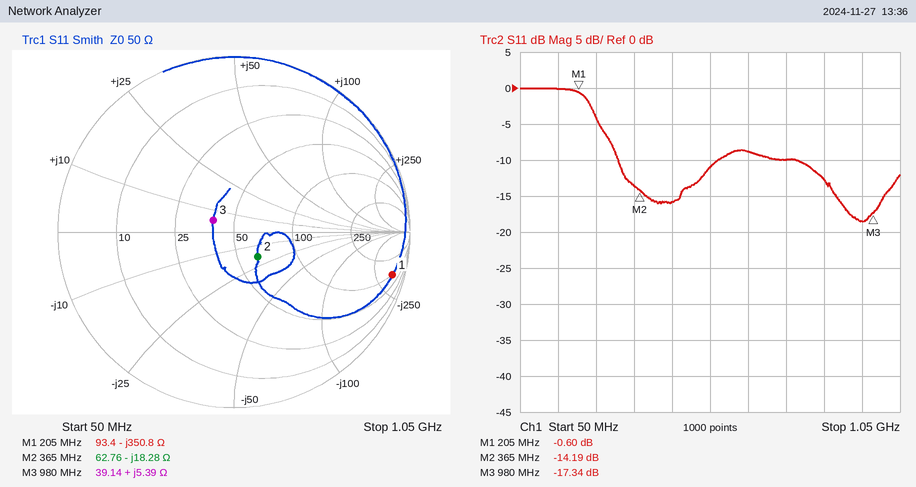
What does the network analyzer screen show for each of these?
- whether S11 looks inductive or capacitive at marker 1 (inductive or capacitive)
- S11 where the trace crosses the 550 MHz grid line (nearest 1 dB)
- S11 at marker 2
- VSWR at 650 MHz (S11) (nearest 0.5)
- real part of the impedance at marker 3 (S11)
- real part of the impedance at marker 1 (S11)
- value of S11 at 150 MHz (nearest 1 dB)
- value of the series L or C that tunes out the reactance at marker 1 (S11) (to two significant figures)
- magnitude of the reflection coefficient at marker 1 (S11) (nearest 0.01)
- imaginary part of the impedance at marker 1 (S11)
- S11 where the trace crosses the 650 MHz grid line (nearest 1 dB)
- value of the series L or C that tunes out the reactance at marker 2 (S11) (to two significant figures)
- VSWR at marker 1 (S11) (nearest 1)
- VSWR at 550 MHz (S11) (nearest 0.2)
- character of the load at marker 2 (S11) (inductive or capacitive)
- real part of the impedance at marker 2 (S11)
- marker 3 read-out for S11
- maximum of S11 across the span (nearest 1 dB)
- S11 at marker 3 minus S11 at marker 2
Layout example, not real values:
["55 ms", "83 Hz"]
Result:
["capacitive", "-11 dB", "-14.19 dB", "2.0", "39.14 Ω", "93.4 Ω", "0 dB", "270 nH", "0.93", "-350.8 Ω", "-9 dB", "8.0 nH", "29", "1.8", "capacitive", "62.76 Ω", "-17.34 dB", "0 dB", "-3.15 dB"]
